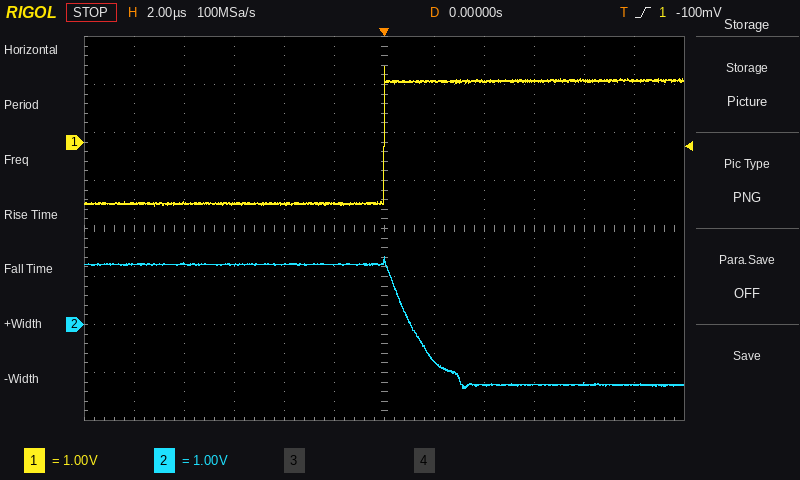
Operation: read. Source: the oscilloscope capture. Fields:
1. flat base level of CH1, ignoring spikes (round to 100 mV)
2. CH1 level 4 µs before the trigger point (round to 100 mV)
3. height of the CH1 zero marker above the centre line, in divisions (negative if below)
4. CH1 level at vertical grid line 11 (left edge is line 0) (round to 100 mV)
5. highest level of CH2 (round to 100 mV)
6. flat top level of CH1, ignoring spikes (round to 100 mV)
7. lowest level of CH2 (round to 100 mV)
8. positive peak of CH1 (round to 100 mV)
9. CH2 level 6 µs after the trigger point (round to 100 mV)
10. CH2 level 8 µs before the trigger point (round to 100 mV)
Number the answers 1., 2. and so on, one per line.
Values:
1. -1.3 V
2. -1.3 V
3. +1.8 div
4. 1.3 V
5. 1.4 V
6. 1.3 V
7. -1.3 V
8. 1.6 V
9. -1.3 V
10. 1.3 V
